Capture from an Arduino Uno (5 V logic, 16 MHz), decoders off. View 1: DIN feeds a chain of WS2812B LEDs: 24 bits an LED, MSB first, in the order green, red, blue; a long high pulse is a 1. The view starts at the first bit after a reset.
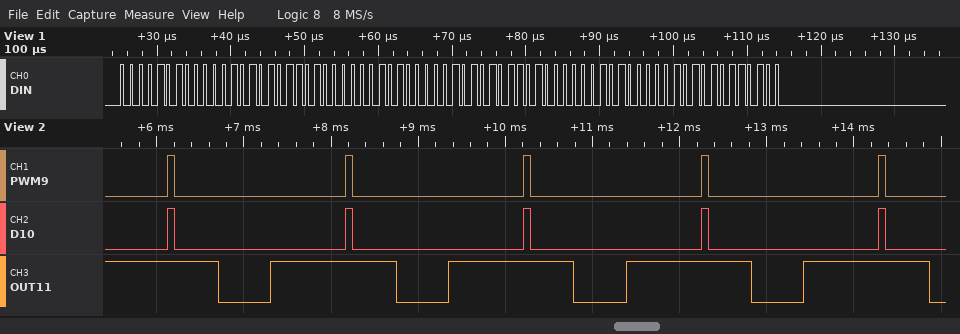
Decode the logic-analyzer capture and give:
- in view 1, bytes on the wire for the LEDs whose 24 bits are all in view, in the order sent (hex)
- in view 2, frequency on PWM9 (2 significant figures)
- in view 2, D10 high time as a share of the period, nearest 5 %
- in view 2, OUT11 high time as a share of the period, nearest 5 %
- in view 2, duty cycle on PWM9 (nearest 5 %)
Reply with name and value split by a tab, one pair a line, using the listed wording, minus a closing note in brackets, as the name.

in view 1, bytes on the wire for the LEDs whose 24 bits are all in view, in the order sent	0A 0A B4 0A 0A B4 0A 0A B4
in view 2, frequency on PWM9	490 Hz
in view 2, D10 high time as a share of the period, nearest 5 %	5 %
in view 2, OUT11 high time as a share of the period, nearest 5 %	70 %
in view 2, duty cycle on PWM9	5 %
